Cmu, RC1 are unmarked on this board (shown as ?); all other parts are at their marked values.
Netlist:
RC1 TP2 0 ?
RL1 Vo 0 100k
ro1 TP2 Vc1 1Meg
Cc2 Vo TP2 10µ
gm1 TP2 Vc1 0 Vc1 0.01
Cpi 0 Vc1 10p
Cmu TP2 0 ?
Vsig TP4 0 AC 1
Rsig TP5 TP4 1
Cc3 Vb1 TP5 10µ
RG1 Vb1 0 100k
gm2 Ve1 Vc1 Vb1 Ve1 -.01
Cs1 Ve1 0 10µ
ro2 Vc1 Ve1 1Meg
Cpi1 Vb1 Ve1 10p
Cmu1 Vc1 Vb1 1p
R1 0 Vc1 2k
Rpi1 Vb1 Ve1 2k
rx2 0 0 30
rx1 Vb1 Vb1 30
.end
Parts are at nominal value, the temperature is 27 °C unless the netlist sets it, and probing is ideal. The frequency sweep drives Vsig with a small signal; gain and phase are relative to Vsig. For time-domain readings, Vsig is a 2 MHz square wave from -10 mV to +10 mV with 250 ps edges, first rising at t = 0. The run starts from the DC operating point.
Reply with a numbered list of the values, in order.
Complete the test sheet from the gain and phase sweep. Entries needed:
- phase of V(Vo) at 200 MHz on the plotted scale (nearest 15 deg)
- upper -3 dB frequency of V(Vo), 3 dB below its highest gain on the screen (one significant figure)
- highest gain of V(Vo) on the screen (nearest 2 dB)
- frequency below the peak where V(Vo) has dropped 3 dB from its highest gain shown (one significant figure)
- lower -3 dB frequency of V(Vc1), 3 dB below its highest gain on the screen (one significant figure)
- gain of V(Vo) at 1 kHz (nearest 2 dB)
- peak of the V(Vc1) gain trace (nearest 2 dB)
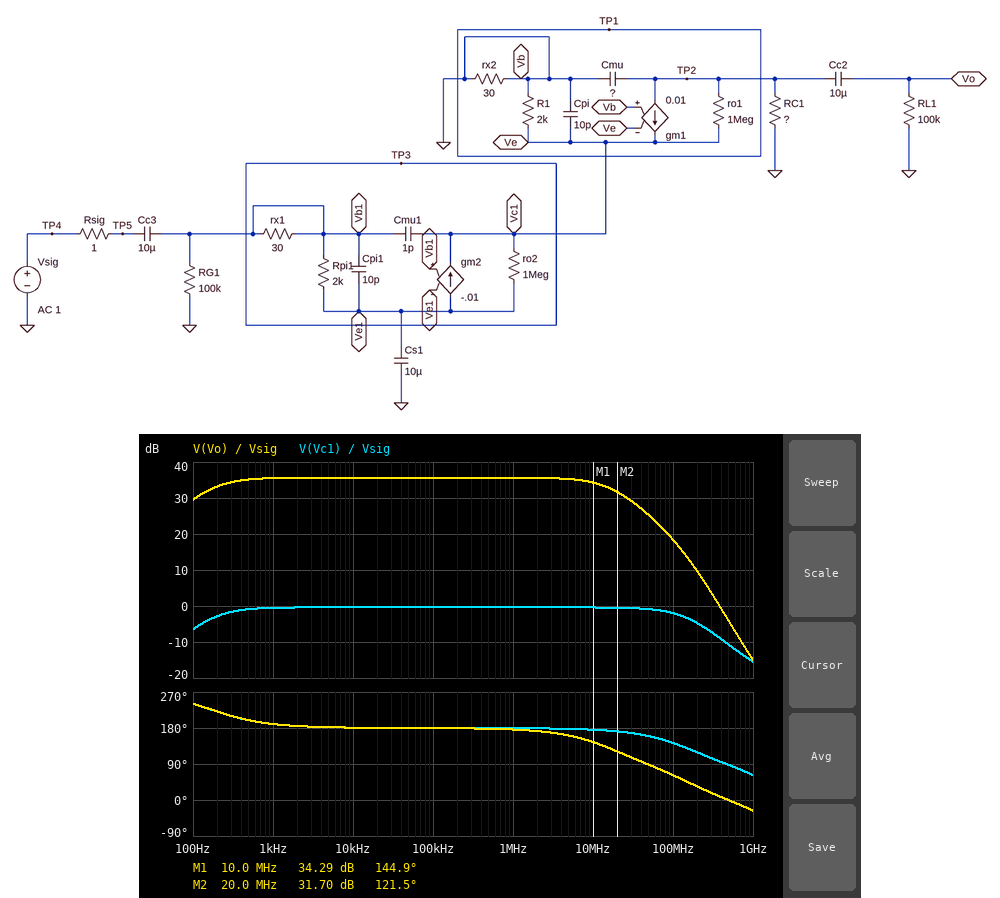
1. 30 deg
2. 20 MHz
3. 36 dB
4. 200 Hz
5. 200 Hz
6. 36 dB
7. 0 dB
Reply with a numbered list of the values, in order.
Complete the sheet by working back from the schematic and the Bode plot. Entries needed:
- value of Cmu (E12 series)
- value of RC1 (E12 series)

1. 1.5 pF
2. 6.8 kΩ
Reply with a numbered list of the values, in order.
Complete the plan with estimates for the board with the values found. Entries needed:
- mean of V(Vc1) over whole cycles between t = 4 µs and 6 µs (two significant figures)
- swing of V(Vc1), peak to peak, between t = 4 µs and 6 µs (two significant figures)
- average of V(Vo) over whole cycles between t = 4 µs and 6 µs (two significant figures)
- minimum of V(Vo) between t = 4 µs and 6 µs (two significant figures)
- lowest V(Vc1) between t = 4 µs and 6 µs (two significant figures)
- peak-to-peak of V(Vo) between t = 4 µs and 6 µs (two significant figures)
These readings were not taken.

1. -9.5 mV
2. 20 mV
3. -600 mV
4. -1.2 V
5. -19 mV
6. 1.2 V
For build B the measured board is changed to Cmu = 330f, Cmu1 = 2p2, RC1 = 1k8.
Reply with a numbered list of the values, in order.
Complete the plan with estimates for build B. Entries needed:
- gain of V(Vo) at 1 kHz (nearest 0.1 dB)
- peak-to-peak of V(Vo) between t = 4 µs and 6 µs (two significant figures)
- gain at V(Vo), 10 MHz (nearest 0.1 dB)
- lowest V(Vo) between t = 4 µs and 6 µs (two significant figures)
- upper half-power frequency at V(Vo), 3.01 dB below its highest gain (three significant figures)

1. 24.4 dB
2. 350 mV
3. 24.5 dB
4. -340 mV
5. 117 MHz
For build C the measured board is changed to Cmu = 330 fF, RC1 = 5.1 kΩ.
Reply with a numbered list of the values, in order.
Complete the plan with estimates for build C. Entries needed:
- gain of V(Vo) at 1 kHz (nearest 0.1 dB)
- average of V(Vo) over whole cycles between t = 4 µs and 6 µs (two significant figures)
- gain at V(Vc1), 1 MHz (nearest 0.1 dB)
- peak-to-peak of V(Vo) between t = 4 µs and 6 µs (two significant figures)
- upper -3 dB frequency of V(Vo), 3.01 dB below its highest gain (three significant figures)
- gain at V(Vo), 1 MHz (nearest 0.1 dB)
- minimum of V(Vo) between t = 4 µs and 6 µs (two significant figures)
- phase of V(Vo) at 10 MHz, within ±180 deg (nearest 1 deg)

1. 33.2 dB
2. -460 mV
3. -0.4 dB
4. 930 mV
5. 76.6 MHz
6. 33.3 dB
7. -920 mV
8. 170 deg
